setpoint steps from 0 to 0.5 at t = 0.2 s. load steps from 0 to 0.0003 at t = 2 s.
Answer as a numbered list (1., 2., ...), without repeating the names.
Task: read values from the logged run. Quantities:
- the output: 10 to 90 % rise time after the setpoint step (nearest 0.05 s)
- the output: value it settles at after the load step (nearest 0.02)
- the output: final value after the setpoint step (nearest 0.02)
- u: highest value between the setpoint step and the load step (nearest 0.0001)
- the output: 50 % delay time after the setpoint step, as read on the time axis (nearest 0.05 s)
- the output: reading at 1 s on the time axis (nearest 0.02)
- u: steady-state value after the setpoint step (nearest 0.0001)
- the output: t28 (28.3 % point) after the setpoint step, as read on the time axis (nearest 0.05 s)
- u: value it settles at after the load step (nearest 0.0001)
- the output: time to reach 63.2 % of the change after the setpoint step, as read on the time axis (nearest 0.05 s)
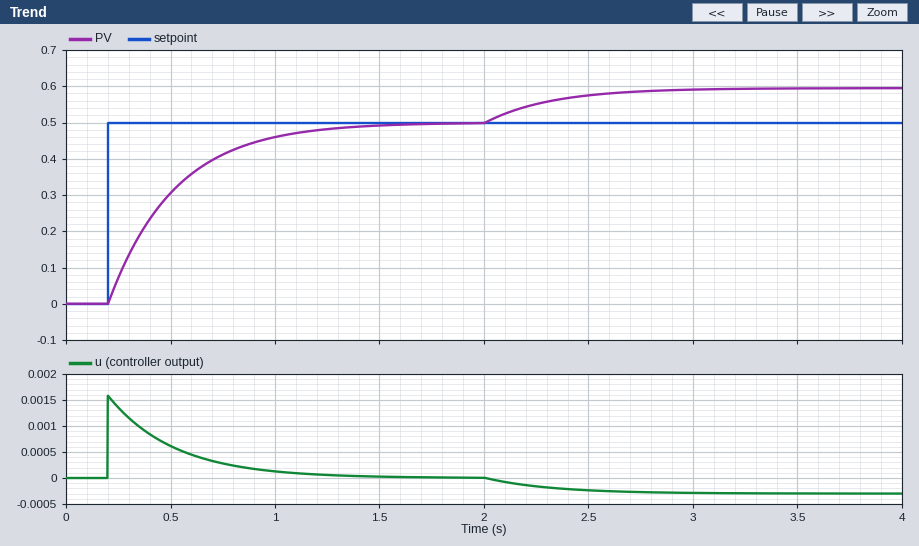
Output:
1. 0.70 s
2. 0.60
3. 0.50
4. 0.0016
5. 0.40 s
6. 0.46
7. 0.0000
8. 0.30 s
9. -0.0003
10. 0.50 s
